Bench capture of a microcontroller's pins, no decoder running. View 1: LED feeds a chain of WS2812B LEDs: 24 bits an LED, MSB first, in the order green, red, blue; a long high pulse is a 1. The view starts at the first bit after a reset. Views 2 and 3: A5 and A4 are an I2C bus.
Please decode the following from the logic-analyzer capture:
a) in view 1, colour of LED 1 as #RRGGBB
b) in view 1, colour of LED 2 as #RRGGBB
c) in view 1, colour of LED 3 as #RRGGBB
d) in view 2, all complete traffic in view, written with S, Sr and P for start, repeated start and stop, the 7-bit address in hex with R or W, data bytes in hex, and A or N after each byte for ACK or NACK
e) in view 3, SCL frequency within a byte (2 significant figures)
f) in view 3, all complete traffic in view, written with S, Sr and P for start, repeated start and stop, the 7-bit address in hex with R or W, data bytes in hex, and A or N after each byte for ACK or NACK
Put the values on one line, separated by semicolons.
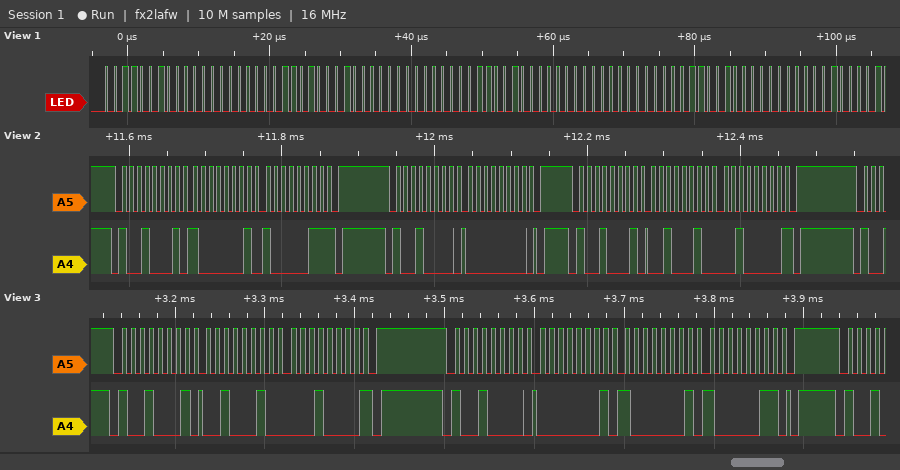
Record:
#00320D; #001032; #000032; S 48R A 81 A 83 N P S 48W A 00 A P S 48R A 22 A 20 N P; 100 kHz; S 48R A 22 A 10 N P S 48W A 01 A 81 A 83 A P
